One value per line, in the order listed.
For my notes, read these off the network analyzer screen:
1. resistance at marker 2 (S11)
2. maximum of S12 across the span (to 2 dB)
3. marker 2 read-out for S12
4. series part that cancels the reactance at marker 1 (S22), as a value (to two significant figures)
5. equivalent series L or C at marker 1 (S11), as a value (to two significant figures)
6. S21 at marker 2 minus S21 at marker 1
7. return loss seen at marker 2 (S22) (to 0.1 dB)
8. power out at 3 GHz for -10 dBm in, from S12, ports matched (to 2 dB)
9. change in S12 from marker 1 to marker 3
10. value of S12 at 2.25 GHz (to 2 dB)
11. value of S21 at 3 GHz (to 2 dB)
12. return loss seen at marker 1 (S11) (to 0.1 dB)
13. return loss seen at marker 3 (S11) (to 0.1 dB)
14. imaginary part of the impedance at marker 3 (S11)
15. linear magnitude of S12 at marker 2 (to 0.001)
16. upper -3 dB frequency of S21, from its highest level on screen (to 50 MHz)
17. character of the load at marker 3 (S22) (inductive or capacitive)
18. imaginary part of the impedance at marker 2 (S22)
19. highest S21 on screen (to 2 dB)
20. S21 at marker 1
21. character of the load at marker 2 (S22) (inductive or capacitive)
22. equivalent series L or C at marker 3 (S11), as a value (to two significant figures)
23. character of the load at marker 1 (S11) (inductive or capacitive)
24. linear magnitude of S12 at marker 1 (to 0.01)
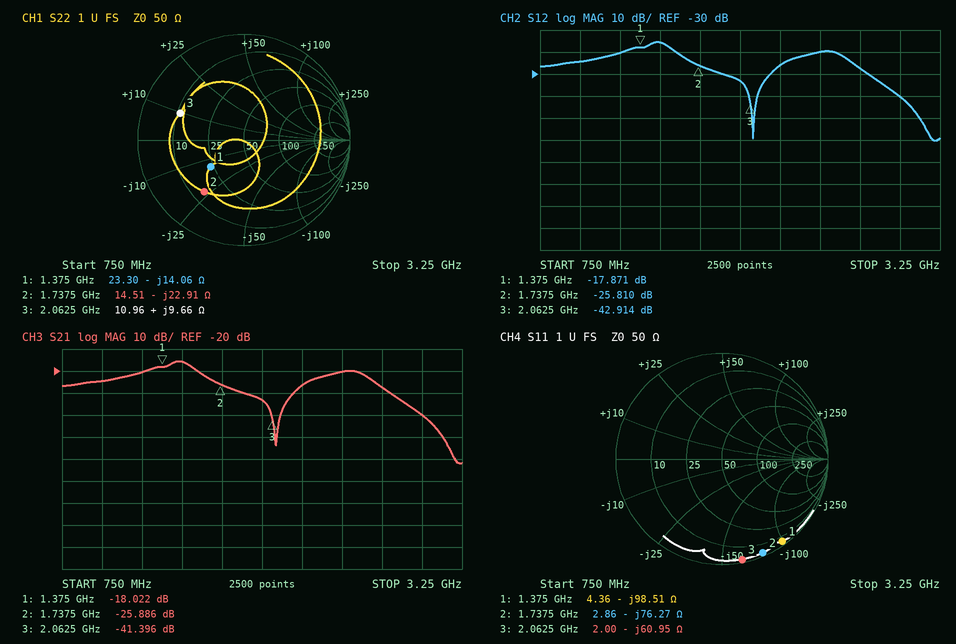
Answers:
2.86 Ω
-16 dB
-25.810 dB
1.6 nH
1.2 pF
-7.864 dB
4.2 dB
-50 dBm
-25.043 dB
-26 dB
-40 dB
0.3 dB
0.3 dB
-60.95 Ω
0.051
1.55 GHz
inductive
-22.91 Ω
-16 dB
-18.022 dB
capacitive
1.3 pF
capacitive
0.13
